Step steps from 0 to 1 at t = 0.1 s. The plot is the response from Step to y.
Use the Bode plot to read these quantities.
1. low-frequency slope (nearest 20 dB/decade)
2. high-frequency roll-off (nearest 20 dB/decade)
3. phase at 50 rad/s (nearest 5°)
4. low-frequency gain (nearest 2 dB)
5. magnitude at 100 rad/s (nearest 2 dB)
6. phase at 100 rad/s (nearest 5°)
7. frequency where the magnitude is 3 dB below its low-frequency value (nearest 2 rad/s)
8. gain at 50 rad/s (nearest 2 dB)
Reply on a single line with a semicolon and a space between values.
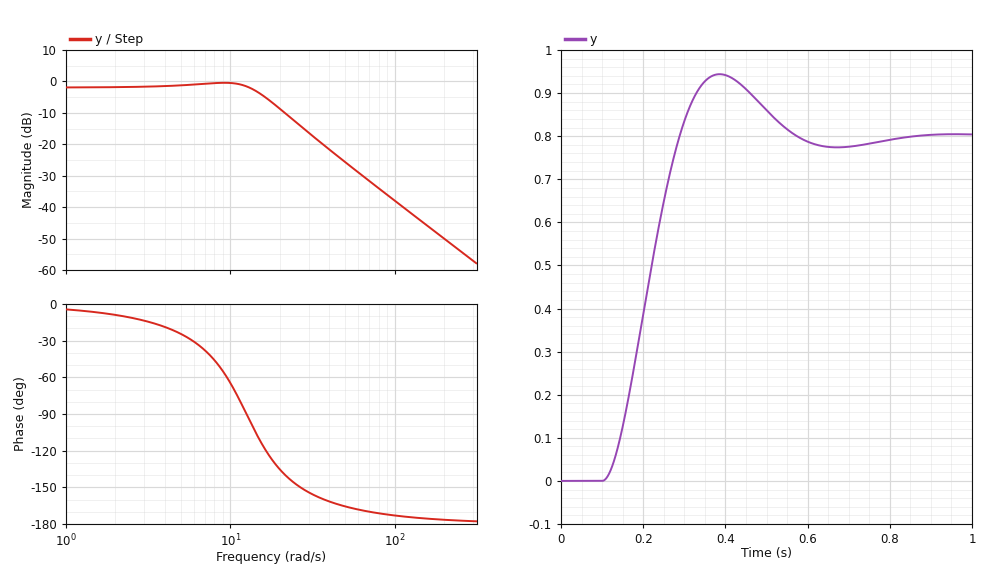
0 dB/decade; -40 dB/decade; -165°; -2 dB; -38 dB; -175°; 16 rad/s; -26 dB
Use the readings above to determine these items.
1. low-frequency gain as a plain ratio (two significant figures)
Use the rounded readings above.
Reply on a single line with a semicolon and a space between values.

0.79
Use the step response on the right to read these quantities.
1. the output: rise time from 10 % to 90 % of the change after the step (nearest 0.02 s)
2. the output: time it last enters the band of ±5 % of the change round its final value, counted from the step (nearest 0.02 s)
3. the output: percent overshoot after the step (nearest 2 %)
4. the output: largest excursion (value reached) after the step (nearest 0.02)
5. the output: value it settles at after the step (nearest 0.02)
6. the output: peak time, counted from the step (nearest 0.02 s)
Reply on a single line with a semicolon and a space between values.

0.12 s; 0.42 s; 18 %; 0.94; 0.80; 0.28 s
